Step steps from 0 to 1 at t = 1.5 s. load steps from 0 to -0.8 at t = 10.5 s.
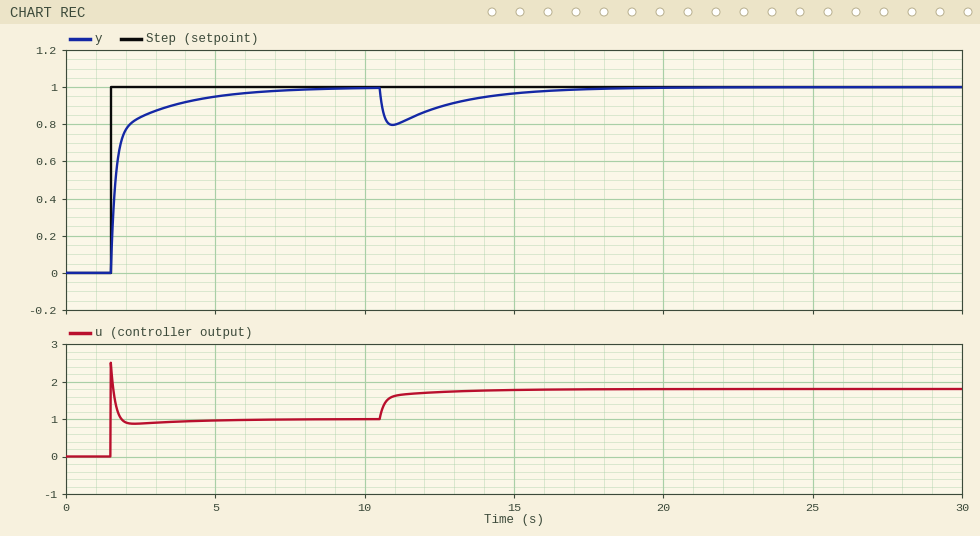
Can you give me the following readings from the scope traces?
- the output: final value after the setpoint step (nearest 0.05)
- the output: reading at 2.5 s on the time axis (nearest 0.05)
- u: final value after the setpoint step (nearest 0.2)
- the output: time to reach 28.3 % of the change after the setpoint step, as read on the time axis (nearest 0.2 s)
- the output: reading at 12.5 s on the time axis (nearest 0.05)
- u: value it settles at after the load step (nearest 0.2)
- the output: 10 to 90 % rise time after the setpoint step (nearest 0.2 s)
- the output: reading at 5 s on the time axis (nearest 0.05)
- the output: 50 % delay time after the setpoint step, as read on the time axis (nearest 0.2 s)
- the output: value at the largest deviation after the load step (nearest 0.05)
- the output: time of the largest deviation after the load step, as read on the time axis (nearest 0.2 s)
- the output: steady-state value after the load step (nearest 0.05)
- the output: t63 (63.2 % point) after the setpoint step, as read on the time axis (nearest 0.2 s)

1.00
0.85
1.0
1.6 s
0.90
1.8
2.0 s
0.95
1.6 s
0.80
11.0 s
1.00
1.8 s
